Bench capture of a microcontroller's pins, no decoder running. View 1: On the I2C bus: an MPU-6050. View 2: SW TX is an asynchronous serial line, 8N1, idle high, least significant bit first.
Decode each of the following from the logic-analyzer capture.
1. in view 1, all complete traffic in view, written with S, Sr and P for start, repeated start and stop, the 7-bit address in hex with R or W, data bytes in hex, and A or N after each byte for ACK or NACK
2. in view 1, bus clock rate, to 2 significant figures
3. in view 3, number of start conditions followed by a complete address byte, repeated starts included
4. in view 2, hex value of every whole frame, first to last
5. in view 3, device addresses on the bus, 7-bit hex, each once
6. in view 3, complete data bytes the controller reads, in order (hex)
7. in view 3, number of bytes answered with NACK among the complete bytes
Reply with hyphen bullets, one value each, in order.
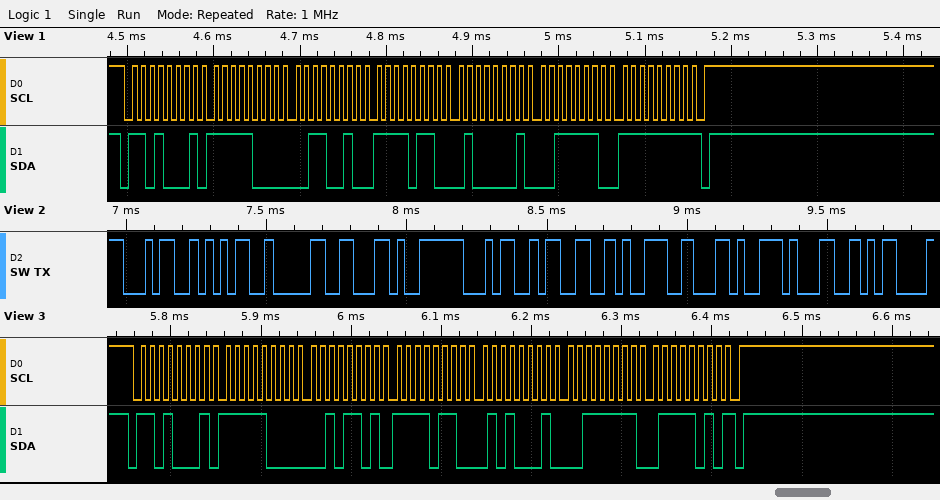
- S 68R A F8 A 32 A F6 A 41 A 3E A FF N P
- 100 kHz
- 1
- 0x34 0x35 0x30 0x2C 0x34 0x33 0x39 0x2C 0x31 0x0D
- 0x68
- F8 2D F6 51 3F 7A
- 1
